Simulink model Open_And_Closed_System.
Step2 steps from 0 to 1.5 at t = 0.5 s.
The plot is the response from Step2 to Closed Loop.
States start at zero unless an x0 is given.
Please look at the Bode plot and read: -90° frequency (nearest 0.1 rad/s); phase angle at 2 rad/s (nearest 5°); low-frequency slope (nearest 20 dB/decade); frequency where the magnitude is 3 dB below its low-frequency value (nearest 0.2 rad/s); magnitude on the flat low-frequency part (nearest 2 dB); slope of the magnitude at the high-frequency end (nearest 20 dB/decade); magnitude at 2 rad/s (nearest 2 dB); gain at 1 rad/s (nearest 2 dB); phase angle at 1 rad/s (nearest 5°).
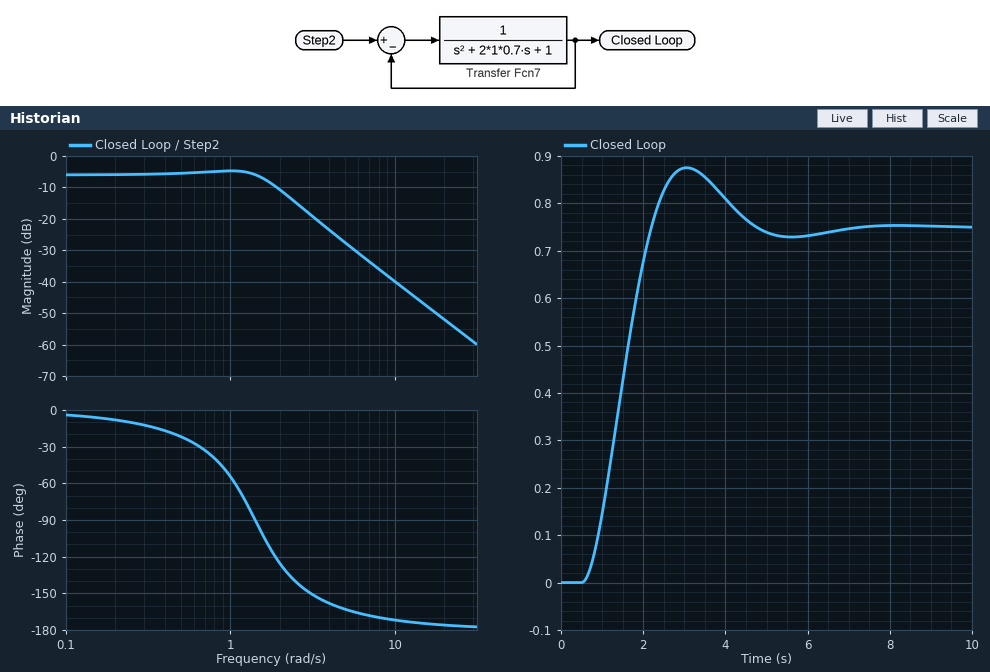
1.4 rad/s
-125°
0 dB/decade
1.8 rad/s
-6 dB
-40 dB/decade
-10 dB
-4 dB
-55°
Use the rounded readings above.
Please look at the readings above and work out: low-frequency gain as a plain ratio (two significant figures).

0.50
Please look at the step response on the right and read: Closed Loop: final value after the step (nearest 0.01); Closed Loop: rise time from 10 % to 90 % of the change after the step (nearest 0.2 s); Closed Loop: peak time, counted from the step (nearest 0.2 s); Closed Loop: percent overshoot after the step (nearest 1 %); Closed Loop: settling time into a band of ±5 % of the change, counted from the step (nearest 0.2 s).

0.75
1.2 s
2.6 s
17 %
3.8 s
